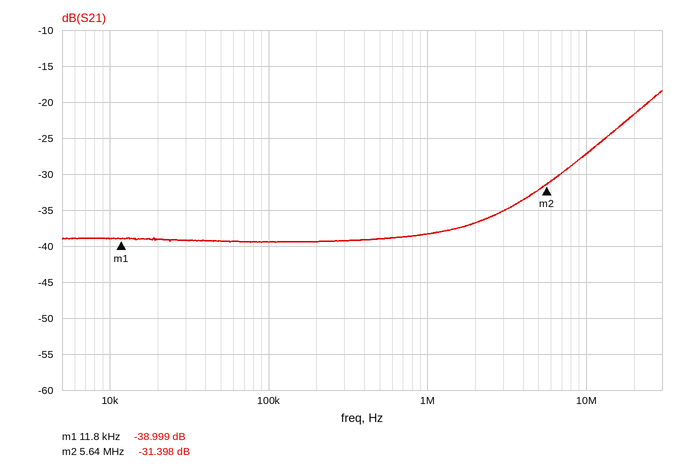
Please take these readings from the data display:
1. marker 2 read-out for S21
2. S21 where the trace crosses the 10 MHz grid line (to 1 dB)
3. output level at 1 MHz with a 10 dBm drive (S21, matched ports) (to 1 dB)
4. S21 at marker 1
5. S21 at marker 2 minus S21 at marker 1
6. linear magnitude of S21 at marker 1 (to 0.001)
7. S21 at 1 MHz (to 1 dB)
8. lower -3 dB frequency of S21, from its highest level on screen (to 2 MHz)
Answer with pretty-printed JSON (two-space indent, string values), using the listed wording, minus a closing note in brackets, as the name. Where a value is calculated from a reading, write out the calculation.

{
  "marker 2 read-out for S21": "-31.398 dB",
  "S21 where the trace crosses the 10 MHz grid line": "-27 dB",
  "output level at 1 MHz with a 10 dBm drive (S21, matched ports)": "10 dBm + (-38 dB) = -28 dBm",
  "S21 at marker 1": "-38.999 dB",
  "S21 at marker 2 minus S21 at marker 1": "-31.398 − (-38.999) = 7.601 dB",
  "linear magnitude of S21 at marker 1": "10^(-38.999/20) ≈ 0.011",
  "S21 at 1 MHz": "-38 dB",
  "lower -3 dB frequency of S21, from its highest level on screen": "20 MHz"
}
